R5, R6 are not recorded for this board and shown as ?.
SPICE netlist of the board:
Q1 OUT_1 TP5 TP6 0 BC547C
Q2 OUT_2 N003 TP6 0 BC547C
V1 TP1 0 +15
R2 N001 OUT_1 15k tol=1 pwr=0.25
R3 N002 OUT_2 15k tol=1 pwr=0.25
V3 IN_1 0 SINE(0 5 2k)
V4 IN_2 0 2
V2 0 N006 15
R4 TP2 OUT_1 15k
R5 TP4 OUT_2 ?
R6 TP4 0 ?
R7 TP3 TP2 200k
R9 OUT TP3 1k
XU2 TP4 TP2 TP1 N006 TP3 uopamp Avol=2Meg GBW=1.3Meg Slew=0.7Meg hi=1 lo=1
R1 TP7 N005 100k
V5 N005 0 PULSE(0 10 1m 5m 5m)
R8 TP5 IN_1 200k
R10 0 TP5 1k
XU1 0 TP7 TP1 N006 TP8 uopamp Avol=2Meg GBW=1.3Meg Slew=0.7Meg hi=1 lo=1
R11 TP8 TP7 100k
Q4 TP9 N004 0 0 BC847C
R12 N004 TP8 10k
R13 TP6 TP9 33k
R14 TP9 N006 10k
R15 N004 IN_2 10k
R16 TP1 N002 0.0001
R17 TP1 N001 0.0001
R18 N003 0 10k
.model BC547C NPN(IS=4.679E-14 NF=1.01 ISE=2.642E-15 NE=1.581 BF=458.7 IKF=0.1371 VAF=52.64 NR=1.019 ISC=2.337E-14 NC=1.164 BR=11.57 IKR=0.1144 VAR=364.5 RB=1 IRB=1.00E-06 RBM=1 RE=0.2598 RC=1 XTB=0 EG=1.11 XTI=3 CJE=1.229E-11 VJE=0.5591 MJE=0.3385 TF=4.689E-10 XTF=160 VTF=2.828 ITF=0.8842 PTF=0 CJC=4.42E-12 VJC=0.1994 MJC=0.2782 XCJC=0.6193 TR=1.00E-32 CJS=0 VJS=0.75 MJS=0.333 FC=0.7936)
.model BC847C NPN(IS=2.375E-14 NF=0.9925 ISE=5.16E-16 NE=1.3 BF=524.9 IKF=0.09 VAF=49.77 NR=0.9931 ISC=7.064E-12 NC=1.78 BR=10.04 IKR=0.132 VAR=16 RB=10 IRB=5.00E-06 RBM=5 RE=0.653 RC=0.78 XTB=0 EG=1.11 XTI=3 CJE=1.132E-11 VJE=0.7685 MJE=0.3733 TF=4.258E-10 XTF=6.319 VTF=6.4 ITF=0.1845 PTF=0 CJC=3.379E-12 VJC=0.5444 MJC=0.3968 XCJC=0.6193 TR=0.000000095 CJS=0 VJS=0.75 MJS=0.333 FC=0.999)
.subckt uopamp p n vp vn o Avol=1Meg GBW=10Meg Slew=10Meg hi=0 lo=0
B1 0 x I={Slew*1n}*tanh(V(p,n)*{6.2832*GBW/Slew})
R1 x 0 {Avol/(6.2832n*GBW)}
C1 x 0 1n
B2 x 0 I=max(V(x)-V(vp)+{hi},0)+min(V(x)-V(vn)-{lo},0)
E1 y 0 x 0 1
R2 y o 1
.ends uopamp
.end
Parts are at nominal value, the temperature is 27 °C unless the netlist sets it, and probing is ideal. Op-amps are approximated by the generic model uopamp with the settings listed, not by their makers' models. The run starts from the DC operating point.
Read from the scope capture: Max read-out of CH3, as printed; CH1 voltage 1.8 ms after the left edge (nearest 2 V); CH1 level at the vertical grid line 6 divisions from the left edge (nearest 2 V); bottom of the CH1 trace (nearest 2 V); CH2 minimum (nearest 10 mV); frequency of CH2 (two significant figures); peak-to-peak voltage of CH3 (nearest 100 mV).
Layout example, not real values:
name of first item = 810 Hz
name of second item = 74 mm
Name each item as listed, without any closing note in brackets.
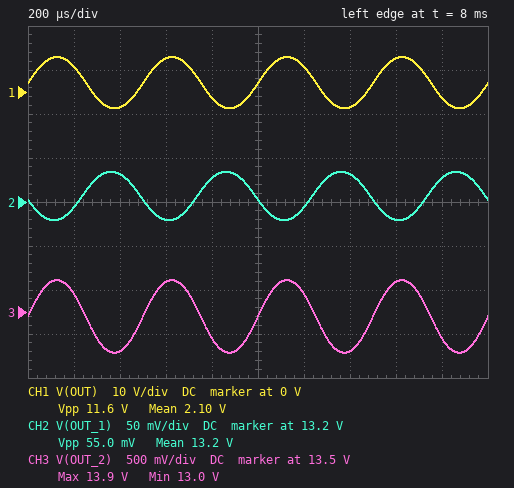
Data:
Max read-out of CH3, as printed = 13.9 V
CH1 voltage 1.8 ms after the left edge = -2 V
CH1 level at the vertical grid line 6 divisions from the left edge = 6 V
bottom of the CH1 trace = -4 V
CH2 minimum = 13.18 V
frequency of CH2 = 2.0 kHz
peak-to-peak voltage of CH3 = 800 mV
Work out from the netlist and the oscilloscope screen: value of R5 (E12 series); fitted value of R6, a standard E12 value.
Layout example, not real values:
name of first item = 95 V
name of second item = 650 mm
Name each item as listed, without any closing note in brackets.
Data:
value of R5 = 27 kΩ
fitted value of R6, a standard E12 value = 330 kΩ
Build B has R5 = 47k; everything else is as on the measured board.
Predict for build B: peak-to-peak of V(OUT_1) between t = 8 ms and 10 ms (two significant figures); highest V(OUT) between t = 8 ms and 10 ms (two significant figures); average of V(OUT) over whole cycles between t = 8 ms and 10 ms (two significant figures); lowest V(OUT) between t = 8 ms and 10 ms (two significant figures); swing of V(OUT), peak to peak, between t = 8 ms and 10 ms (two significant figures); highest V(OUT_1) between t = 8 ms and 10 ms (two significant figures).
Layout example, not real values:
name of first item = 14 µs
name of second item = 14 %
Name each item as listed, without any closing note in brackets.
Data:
peak-to-peak of V(OUT_1) between t = 8 ms and 10 ms = 74 mV
highest V(OUT) between t = 8 ms and 10 ms = 2.9 V
average of V(OUT) over whole cycles between t = 8 ms and 10 ms = -2.8 V
lowest V(OUT) between t = 8 ms and 10 ms = -8.5 V
swing of V(OUT), peak to peak, between t = 8 ms and 10 ms = 11 V
highest V(OUT_1) between t = 8 ms and 10 ms = 13 V
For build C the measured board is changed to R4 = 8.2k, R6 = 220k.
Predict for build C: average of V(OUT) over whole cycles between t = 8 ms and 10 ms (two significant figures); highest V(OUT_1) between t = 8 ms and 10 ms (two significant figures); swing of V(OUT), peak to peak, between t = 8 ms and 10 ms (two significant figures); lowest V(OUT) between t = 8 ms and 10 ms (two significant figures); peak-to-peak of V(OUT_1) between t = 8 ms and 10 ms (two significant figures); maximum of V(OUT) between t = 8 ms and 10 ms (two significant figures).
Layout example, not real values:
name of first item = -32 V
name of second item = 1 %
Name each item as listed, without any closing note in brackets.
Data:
average of V(OUT) over whole cycles between t = 8 ms and 10 ms = -7.3 V
highest V(OUT_1) between t = 8 ms and 10 ms = 13 V
swing of V(OUT), peak to peak, between t = 8 ms and 10 ms = 14 V
lowest V(OUT) between t = 8 ms and 10 ms = -14 V
peak-to-peak of V(OUT_1) between t = 8 ms and 10 ms = 150 mV
maximum of V(OUT) between t = 8 ms and 10 ms = -140 mV
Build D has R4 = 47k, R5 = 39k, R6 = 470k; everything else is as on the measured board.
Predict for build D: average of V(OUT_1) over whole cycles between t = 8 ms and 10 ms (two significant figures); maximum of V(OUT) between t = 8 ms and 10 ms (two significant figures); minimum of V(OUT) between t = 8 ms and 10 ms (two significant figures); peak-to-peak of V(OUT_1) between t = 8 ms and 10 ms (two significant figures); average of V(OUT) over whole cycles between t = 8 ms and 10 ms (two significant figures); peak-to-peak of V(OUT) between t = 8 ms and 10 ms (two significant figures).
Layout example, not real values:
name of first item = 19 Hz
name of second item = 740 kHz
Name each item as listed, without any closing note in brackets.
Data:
average of V(OUT_1) over whole cycles between t = 8 ms and 10 ms = 14 V
maximum of V(OUT) between t = 8 ms and 10 ms = 11 V
minimum of V(OUT) between t = 8 ms and 10 ms = 5.0 V
peak-to-peak of V(OUT_1) between t = 8 ms and 10 ms = 470 mV
average of V(OUT) over whole cycles between t = 8 ms and 10 ms = 8.0 V
peak-to-peak of V(OUT) between t = 8 ms and 10 ms = 6.0 V
